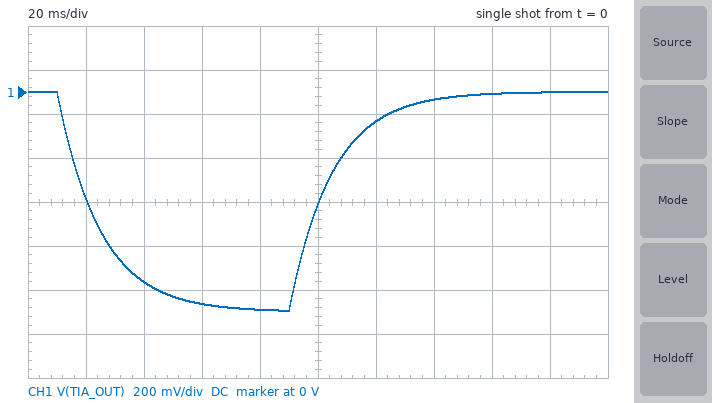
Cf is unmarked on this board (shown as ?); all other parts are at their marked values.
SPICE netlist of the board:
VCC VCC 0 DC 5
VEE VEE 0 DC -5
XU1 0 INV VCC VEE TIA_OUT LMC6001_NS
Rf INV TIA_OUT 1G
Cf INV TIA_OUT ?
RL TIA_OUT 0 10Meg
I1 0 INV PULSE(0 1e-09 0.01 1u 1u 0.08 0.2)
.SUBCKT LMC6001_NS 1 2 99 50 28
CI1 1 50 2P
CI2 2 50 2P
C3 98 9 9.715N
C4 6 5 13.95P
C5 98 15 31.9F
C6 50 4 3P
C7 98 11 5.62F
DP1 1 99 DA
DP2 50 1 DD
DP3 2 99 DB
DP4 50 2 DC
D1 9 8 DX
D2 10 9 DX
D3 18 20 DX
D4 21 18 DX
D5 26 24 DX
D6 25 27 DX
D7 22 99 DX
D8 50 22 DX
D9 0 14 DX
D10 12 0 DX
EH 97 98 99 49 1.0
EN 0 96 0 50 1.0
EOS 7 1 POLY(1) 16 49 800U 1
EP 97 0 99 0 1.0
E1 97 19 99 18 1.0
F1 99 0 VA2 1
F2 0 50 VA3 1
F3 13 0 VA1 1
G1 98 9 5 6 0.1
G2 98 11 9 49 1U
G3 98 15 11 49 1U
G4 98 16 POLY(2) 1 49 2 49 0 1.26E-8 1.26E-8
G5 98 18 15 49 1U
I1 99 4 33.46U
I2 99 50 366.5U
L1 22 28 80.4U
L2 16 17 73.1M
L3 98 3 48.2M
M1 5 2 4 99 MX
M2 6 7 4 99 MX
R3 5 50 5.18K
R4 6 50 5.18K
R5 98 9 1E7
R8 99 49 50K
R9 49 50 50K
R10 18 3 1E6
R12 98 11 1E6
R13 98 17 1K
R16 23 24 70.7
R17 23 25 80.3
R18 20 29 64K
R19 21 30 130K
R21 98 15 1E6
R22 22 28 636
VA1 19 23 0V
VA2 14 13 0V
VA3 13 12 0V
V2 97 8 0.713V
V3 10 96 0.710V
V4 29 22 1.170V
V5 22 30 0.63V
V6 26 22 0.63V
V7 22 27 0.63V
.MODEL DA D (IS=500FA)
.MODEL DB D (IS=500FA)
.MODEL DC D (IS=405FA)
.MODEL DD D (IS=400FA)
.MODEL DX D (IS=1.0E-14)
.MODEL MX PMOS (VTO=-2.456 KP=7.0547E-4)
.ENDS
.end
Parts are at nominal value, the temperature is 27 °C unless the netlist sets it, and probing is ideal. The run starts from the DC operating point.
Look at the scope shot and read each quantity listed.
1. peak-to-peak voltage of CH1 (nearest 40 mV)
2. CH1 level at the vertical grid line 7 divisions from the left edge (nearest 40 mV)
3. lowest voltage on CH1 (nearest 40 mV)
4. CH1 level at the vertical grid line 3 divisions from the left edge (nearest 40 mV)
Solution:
1.00 V
-40 mV
-1.00 V
-960 mV
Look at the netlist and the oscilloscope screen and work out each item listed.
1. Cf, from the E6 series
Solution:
15 pF
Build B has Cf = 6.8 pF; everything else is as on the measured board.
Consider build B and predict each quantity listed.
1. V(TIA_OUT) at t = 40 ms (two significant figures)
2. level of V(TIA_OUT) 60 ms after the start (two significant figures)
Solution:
-990 mV
-1.0 V
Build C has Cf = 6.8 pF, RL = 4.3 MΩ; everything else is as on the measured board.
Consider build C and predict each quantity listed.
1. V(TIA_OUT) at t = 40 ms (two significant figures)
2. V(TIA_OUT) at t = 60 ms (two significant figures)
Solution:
-990 mV
-1.0 V
